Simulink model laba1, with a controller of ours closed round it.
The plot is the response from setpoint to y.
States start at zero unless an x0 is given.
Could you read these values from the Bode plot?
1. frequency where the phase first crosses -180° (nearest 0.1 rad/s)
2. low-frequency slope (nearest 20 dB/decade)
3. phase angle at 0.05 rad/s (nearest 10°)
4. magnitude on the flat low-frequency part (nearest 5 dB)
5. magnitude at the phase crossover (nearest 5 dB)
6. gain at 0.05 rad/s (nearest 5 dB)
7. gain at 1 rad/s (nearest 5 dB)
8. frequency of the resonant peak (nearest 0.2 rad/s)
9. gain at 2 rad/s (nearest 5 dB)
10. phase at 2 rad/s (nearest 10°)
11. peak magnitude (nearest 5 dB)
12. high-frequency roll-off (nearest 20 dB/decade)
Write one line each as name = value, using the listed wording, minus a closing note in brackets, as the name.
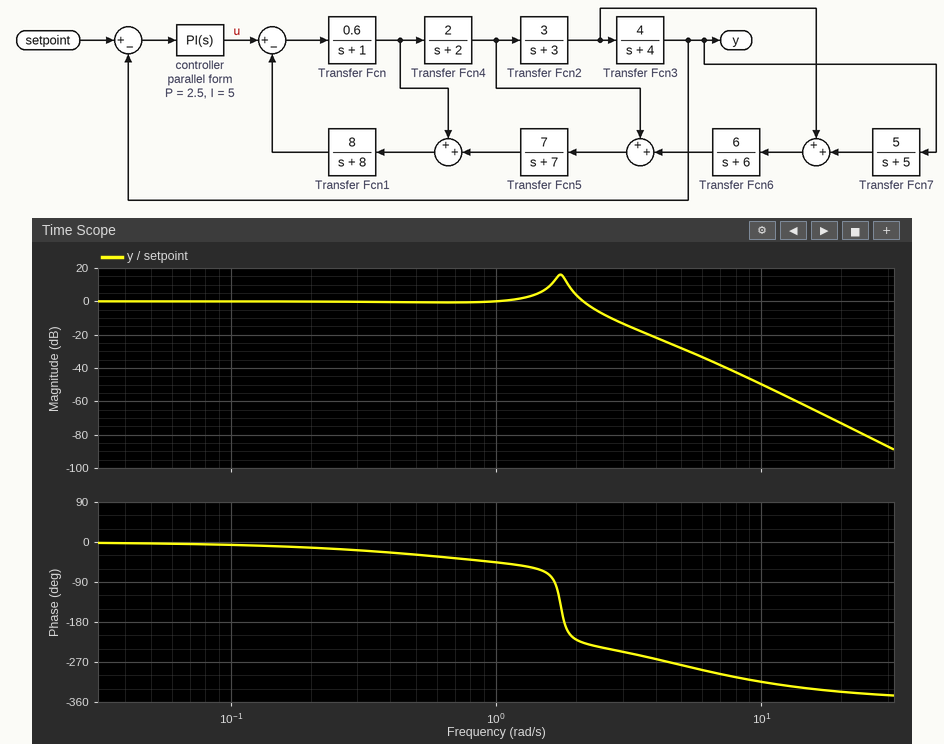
frequency where the phase first crosses -180° = 1.8 rad/s
low-frequency slope = 0 dB/decade
phase angle at 0.05 rad/s = 0°
magnitude on the flat low-frequency part = 0 dB
magnitude at the phase crossover = 15 dB
gain at 0.05 rad/s = 0 dB
gain at 1 rad/s = 0 dB
frequency of the resonant peak = 1.8 rad/s
gain at 2 rad/s = 5 dB
phase at 2 rad/s = -220°
peak magnitude = 15 dB
high-frequency roll-off = -80 dB/decade
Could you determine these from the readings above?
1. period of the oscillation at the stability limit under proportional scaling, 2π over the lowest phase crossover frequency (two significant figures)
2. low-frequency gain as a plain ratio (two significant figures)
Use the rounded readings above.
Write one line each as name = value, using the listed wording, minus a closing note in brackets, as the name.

period of the oscillation at the stability limit under proportional scaling, 2π over the lowest phase crossover frequency = 3.5 s
low-frequency gain as a plain ratio = 1.0
